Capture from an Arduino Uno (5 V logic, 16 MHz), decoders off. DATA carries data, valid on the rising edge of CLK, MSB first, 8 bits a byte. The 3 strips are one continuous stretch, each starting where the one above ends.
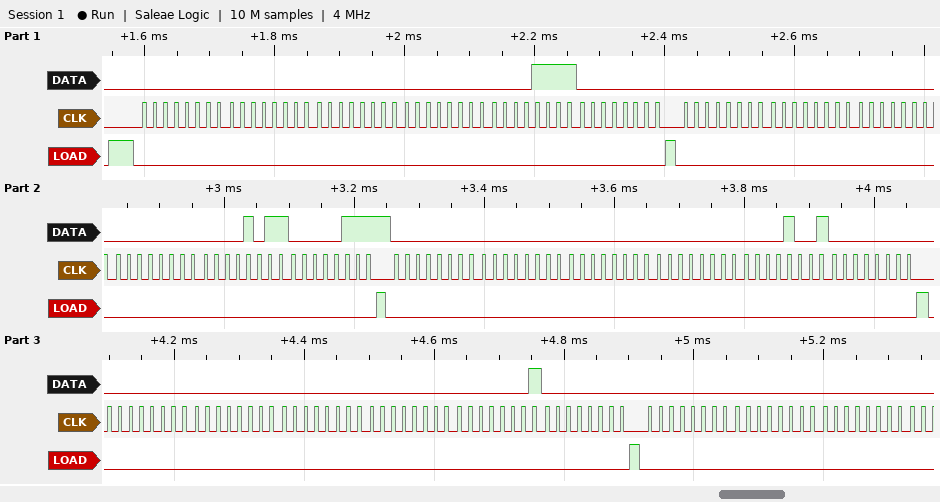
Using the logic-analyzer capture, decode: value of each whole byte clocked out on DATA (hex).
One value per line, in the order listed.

00 00 00 00 0F 00 00 00 00 00 0B 07 00 00 00 00 09 00 00 00 00 00 01 00 00 00 00
